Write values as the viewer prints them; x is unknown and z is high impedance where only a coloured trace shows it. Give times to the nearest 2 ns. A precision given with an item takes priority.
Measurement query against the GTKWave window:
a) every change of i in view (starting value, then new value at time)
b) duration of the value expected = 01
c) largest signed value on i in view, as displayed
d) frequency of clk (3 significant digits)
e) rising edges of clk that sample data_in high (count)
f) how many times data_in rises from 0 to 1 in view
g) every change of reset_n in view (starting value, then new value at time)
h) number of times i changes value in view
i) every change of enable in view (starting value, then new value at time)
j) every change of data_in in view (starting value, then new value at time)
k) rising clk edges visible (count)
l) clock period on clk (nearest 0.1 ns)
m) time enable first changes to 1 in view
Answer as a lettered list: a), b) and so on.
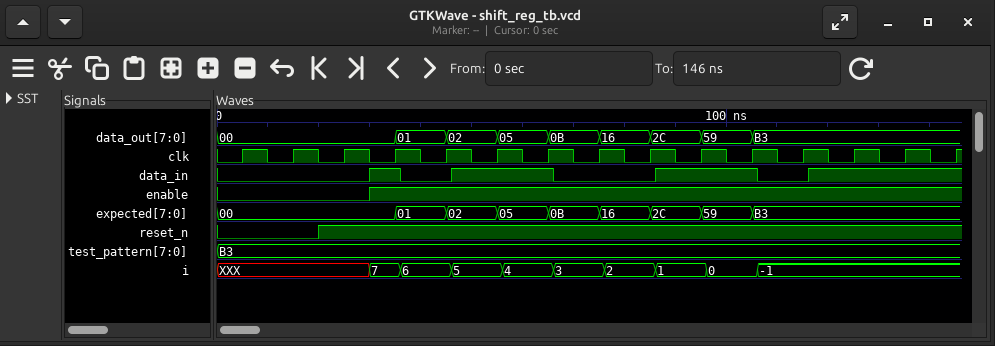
a) XXX, 7 at 30 ns, 6 at 36 ns, 5 at 46 ns, 4 at 56 ns, 3 at 66 ns, 2 at 76 ns, 1 at 86 ns, 0 at 96 ns, -1 at 106 ns
b) 10 ns
c) 7
d) 100 MHz
e) 8
f) 4
g) 0, 1 at 20 ns
h) 9
i) 0, 1 at 30 ns
j) 0, 1 at 30 ns, 0 at 36 ns, 1 at 46 ns, 0 at 66 ns, 1 at 86 ns, 0 at 106 ns, 1 at 116 ns
k) 15
l) 10 ns
m) 30 ns
